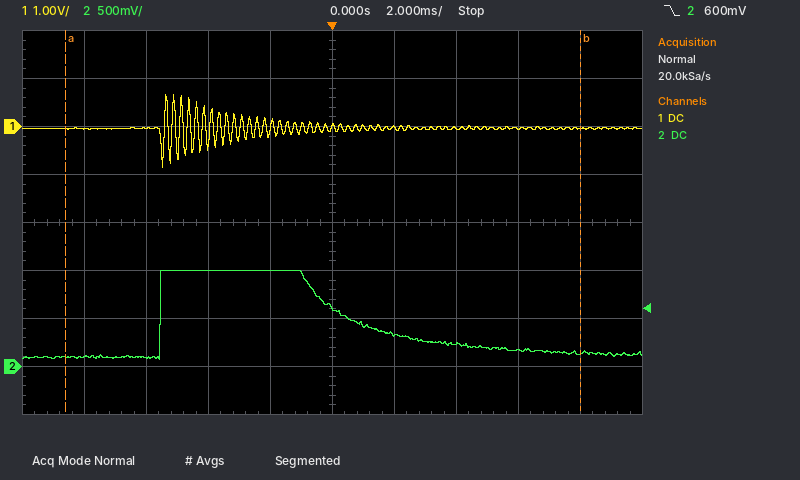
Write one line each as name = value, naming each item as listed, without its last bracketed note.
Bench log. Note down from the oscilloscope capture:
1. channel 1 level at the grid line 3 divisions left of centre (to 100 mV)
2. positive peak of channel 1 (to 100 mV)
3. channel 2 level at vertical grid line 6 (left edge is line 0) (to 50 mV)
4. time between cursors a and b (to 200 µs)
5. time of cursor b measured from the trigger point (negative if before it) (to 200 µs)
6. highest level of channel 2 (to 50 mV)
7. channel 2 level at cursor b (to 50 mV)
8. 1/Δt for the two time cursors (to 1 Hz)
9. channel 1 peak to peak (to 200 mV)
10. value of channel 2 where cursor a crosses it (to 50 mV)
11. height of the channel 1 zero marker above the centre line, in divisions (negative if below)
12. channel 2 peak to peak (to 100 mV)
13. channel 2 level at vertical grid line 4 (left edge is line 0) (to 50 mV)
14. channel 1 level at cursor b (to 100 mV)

channel 1 level at the grid line 3 divisions left of centre = 0.0 V
positive peak of channel 1 = 700 mV
channel 2 level at vertical grid line 6 (left edge is line 0) = 350 mV
time between cursors a and b = 16.6 ms
time of cursor b measured from the trigger point (negative if before it) = +8.0 ms
highest level of channel 2 = 1.00 V
channel 2 level at cursor b = 150 mV
1/Δt for the two time cursors = 60 Hz
channel 1 peak to peak = 1.6 V
value of channel 2 where cursor a crosses it = 100 mV
height of the channel 1 zero marker above the centre line, in divisions = +2.0 div
channel 2 peak to peak = 900 mV
channel 2 level at vertical grid line 4 (left edge is line 0) = 1.00 V
channel 1 level at cursor b = 0.0 V
